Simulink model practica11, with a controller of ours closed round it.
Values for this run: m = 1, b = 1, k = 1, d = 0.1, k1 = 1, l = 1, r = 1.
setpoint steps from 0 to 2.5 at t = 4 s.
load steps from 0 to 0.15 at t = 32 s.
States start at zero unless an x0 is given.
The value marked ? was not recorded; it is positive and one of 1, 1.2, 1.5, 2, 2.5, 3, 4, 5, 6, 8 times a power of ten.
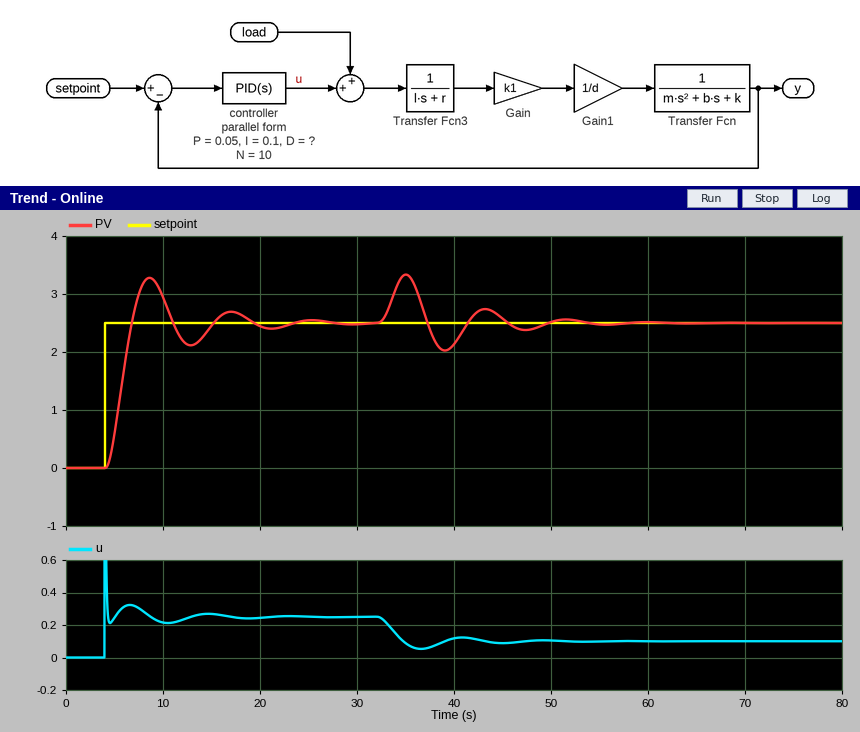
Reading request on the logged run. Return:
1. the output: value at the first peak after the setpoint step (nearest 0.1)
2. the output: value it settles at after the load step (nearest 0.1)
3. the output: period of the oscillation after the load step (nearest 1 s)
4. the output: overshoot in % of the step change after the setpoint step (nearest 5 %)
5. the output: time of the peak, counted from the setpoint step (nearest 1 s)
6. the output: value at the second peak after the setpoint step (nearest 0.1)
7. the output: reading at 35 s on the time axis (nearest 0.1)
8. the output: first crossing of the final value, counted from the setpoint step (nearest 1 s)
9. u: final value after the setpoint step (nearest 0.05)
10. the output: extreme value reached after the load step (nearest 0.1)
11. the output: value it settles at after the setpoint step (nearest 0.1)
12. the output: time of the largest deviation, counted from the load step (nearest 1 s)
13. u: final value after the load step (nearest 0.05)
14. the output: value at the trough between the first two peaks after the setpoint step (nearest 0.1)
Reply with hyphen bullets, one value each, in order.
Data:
- 3.3
- 2.5
- 8 s
- 30 %
- 5 s
- 2.7
- 3.3
- 3 s
- 0.25
- 3.3
- 2.5
- 3 s
- 0.10
- 2.1
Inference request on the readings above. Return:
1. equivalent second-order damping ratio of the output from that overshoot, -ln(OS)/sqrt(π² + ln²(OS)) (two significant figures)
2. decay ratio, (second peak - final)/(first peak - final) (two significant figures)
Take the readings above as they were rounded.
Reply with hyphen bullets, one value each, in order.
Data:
- 0.36
- 0.25
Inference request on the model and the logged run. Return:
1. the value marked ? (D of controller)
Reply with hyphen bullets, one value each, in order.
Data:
- 0.08
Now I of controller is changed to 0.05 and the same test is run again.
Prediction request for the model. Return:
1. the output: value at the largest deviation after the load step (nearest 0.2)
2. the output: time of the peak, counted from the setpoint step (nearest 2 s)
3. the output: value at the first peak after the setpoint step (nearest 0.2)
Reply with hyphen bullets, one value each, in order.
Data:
- 3.4
- 8 s
- 2.6
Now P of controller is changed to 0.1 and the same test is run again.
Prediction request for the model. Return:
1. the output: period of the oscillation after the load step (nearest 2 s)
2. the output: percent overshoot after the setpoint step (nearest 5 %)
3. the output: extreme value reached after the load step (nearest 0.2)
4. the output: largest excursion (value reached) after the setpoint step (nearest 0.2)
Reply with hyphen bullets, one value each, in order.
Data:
- 6 s
- 25 %
- 3.2
- 3.2
